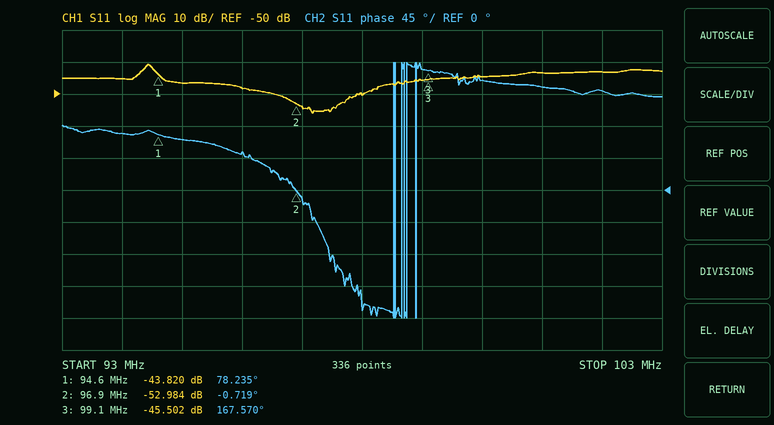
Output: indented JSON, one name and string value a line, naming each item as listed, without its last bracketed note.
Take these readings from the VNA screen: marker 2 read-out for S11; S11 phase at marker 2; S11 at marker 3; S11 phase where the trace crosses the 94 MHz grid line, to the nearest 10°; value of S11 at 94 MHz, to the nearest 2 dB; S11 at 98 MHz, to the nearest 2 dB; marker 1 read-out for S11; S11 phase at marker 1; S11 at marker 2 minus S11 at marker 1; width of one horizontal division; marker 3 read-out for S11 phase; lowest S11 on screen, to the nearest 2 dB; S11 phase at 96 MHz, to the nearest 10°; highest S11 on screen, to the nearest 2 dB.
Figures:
{
  "marker 2 read-out for S11": "-52.984 dB",
  "S11 phase at marker 2": "-0.719°",
  "S11 at marker 3": "-45.502 dB",
  "S11 phase where the trace crosses the 94 MHz grid line, to the nearest 10°": "80°",
  "value of S11 at 94 MHz, to the nearest 2 dB": "-46 dB",
  "S11 at 98 MHz, to the nearest 2 dB": "-50 dB",
  "marker 1 read-out for S11": "-43.820 dB",
  "S11 phase at marker 1": "78.235°",
  "S11 at marker 2 minus S11 at marker 1": "-9.164 dB",
  "width of one horizontal division": "1 MHz",
  "marker 3 read-out for S11 phase": "167.570°",
  "lowest S11 on screen, to the nearest 2 dB": "-56 dB",
  "S11 phase at 96 MHz, to the nearest 10°": "50°",
  "highest S11 on screen, to the nearest 2 dB": "-40 dB"
}
